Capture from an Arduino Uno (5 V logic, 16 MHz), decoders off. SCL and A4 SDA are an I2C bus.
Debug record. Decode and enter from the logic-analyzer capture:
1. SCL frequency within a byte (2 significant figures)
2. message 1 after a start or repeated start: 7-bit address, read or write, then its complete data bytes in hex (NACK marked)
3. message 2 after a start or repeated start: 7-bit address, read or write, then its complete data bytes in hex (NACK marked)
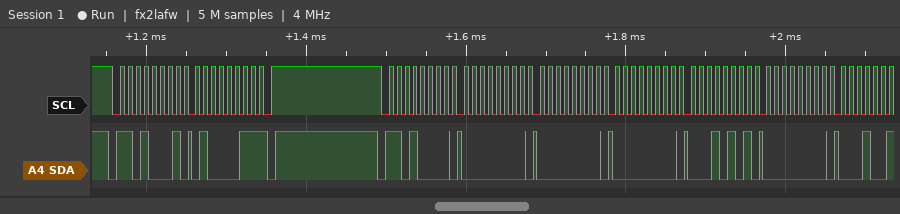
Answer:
100 kHz
0x68 read: 43 NACK
0x68 write: 00 00 00 15 00
